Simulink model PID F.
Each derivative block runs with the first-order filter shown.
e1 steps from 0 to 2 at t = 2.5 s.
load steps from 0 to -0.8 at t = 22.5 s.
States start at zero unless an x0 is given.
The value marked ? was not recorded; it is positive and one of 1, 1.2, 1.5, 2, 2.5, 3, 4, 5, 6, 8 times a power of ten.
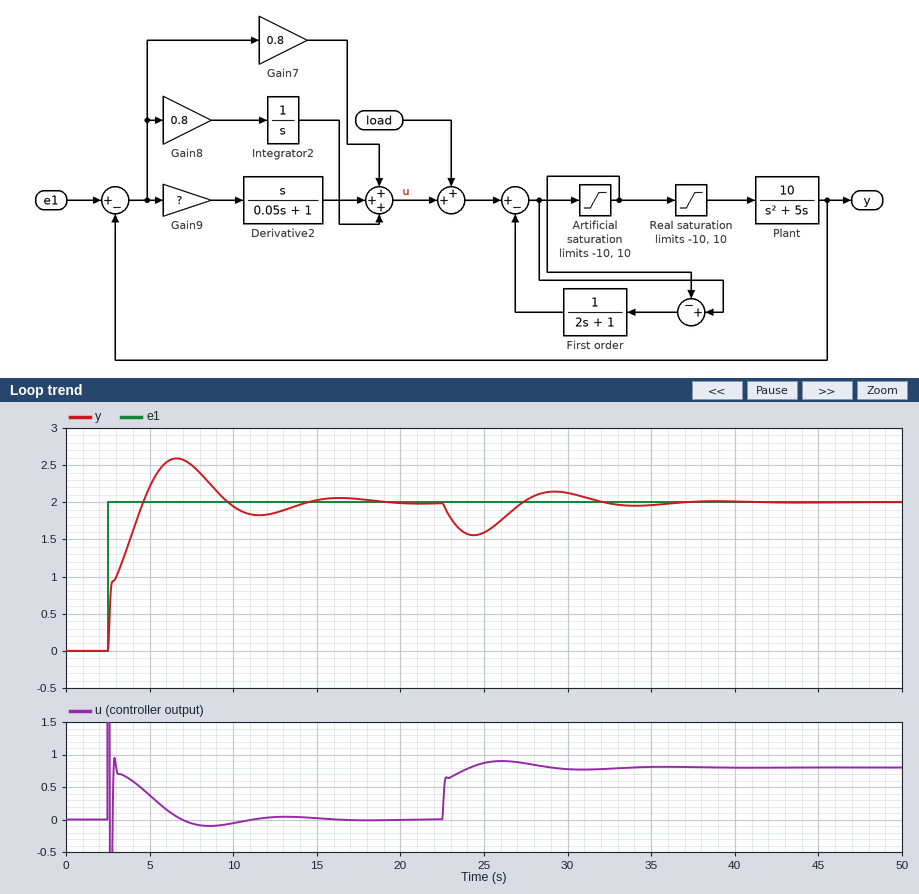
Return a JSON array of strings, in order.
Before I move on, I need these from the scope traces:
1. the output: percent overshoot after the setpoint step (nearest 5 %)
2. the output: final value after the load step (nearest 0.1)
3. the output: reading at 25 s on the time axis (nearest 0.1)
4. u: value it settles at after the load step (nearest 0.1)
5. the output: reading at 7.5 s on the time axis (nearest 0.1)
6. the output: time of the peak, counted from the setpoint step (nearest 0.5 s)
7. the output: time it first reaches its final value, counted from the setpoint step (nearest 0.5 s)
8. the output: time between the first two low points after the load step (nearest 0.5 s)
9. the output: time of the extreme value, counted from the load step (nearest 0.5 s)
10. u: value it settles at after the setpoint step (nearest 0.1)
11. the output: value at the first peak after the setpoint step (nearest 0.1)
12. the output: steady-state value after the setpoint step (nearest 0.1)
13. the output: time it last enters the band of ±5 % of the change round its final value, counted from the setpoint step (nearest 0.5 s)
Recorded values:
["30 %", "2.0", "1.6", "0.8", "2.5", "4.0 s", "2.0 s", "9.5 s", "2.0 s", "0.0", "2.6", "2.0", "10.5 s"]
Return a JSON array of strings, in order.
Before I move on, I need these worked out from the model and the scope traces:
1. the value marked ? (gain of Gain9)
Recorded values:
["1.2"]
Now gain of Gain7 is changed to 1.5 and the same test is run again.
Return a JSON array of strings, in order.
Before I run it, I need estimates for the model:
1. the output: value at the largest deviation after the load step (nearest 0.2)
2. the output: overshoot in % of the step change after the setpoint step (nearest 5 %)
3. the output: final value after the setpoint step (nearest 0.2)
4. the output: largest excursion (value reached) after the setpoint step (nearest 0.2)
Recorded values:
["1.6", "15 %", "2.0", "2.4"]
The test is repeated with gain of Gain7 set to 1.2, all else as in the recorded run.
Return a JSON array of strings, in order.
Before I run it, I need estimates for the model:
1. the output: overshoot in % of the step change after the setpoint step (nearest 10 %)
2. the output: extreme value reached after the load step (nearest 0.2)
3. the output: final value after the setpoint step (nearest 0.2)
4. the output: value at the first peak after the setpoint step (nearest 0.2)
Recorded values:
["20 %", "1.6", "2.0", "2.4"]
